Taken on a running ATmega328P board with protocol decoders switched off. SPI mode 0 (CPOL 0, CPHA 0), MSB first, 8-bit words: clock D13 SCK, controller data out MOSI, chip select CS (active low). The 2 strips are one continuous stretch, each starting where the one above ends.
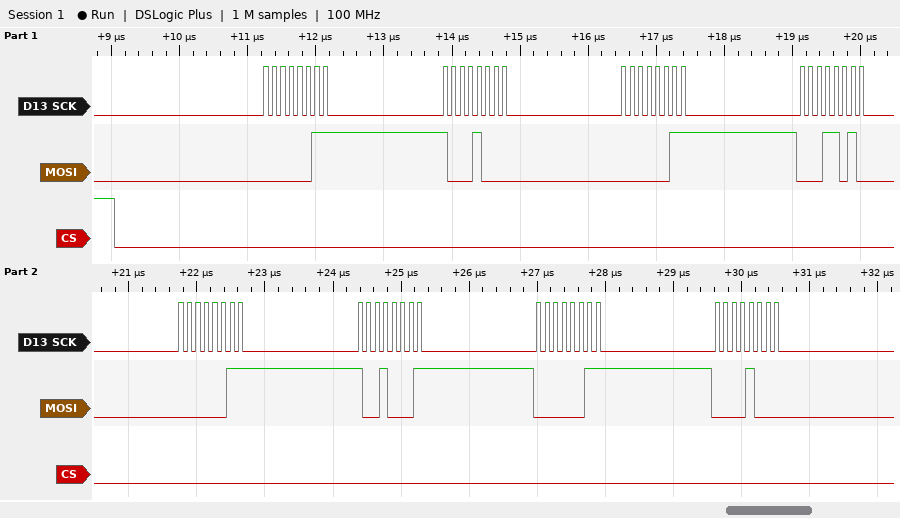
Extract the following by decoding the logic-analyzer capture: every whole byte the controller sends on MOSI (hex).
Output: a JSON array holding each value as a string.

["03 88 03 1A 03 91 03 08"]
